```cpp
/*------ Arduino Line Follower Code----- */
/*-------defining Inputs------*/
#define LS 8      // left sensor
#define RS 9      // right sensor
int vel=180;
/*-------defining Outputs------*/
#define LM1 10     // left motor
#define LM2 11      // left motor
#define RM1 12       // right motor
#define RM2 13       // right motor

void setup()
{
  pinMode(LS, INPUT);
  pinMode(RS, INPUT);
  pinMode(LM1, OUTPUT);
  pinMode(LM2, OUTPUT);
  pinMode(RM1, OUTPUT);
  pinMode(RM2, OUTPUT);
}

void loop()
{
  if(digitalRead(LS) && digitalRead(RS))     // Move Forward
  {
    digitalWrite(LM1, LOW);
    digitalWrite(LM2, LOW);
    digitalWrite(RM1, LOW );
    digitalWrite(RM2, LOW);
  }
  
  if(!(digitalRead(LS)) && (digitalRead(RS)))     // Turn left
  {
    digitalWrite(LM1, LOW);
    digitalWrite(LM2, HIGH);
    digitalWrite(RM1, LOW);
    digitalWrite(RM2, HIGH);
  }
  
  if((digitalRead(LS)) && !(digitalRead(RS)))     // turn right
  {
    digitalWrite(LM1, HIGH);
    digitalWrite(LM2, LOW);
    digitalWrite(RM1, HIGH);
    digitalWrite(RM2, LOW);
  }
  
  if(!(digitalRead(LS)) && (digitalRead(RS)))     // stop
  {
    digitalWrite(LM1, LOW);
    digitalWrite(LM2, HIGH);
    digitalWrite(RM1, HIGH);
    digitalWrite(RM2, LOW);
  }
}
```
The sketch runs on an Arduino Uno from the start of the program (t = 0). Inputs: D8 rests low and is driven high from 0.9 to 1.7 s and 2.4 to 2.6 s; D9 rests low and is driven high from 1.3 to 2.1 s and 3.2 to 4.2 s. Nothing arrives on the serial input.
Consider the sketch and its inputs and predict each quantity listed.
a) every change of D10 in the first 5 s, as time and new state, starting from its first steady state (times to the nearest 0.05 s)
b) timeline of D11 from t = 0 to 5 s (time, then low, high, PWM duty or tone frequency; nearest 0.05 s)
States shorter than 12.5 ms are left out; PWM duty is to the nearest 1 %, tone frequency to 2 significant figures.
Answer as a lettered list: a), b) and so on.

a) 0 s low; 0.9 s high; 1.3 s low; 2.4 s high; 3.2 s low
b) 0 s low; 1.7 s high; 2.4 s low; 3.2 s high
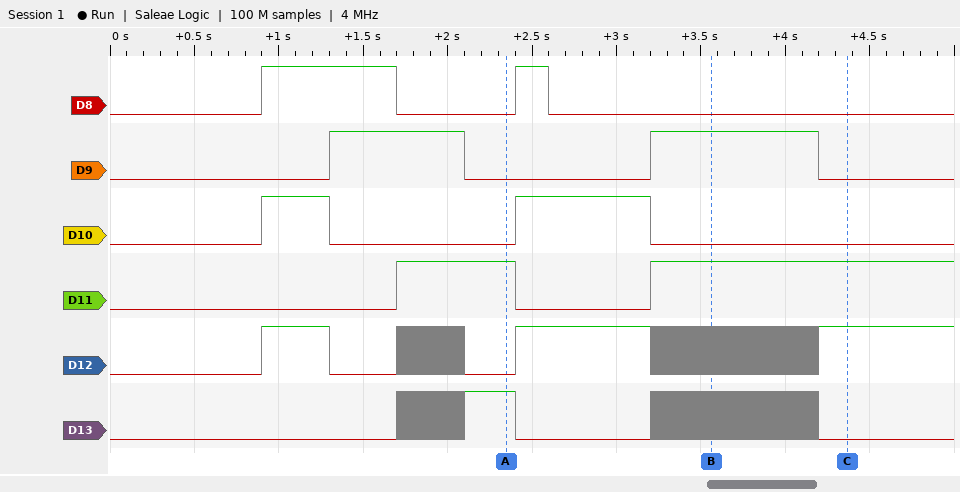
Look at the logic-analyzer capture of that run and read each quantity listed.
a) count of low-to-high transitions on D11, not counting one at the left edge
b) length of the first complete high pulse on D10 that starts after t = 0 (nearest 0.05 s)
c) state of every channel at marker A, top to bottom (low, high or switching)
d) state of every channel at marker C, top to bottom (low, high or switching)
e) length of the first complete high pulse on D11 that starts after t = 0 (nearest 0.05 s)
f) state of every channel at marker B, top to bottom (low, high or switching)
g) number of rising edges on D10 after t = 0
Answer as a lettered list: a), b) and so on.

a) 2
b) 0.40 s
c) D8 low, D9 low, D10 low, D11 high, D12 low, D13 high
d) D8 low, D9 low, D10 low, D11 high, D12 high, D13 low
e) 0.70 s
f) D8 low, D9 high, D10 low, D11 high, D12 switching, D13 switching
g) 2
